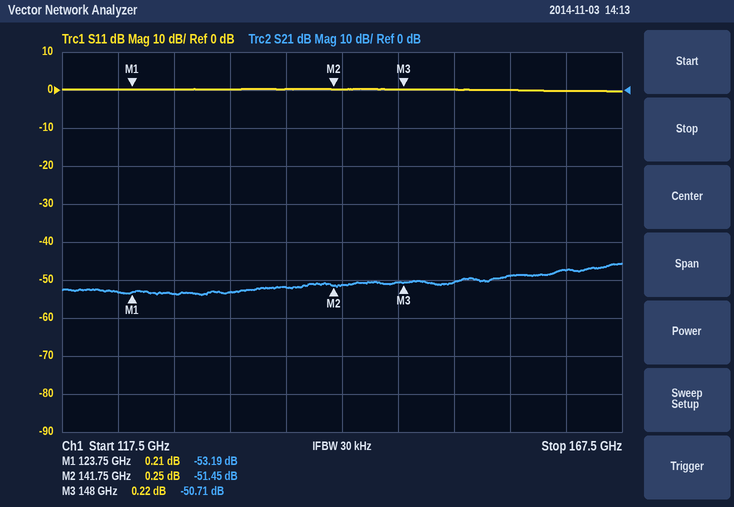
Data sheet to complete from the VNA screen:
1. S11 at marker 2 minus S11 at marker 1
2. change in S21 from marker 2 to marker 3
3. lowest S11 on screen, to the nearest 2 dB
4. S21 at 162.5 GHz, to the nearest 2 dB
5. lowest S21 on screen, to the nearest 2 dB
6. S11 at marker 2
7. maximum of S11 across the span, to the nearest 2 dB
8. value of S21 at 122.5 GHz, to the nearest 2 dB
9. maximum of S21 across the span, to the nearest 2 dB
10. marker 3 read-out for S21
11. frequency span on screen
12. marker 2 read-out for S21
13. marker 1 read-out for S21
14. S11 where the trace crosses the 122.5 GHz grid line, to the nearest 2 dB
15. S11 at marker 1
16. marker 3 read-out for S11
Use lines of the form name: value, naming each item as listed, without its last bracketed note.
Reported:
S11 at marker 2 minus S11 at marker 1: 0.04 dB
change in S21 from marker 2 to marker 3: 0.74 dB
lowest S11 on screen, to the nearest 2 dB: 0 dB
S21 at 162.5 GHz, to the nearest 2 dB: -48 dB
lowest S21 on screen, to the nearest 2 dB: -54 dB
S11 at marker 2: 0.25 dB
maximum of S11 across the span, to the nearest 2 dB: 0 dB
value of S21 at 122.5 GHz, to the nearest 2 dB: -54 dB
maximum of S21 across the span, to the nearest 2 dB: -46 dB
marker 3 read-out for S21: -50.71 dB
frequency span on screen: 50 GHz
marker 2 read-out for S21: -51.45 dB
marker 1 read-out for S21: -53.19 dB
S11 where the trace crosses the 122.5 GHz grid line, to the nearest 2 dB: 0 dB
S11 at marker 1: 0.21 dB
marker 3 read-out for S11: 0.22 dB
